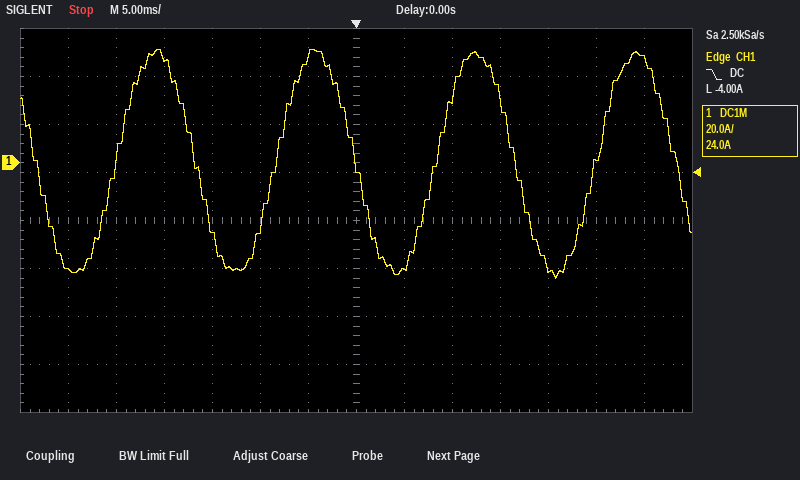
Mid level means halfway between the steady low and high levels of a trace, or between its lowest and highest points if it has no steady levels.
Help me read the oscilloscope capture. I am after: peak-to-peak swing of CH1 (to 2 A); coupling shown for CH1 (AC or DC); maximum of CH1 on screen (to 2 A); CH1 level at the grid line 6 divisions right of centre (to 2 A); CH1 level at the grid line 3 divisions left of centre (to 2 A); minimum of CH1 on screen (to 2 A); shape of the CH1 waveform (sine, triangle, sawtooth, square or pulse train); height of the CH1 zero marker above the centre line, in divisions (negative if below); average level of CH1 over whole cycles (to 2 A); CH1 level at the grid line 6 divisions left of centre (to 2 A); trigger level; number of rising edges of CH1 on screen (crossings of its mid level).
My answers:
96 A
DC
48 A
44 A
-28 A
-48 A
sine
+1.2 div
0 A
-44 A
-4.00 A
4
